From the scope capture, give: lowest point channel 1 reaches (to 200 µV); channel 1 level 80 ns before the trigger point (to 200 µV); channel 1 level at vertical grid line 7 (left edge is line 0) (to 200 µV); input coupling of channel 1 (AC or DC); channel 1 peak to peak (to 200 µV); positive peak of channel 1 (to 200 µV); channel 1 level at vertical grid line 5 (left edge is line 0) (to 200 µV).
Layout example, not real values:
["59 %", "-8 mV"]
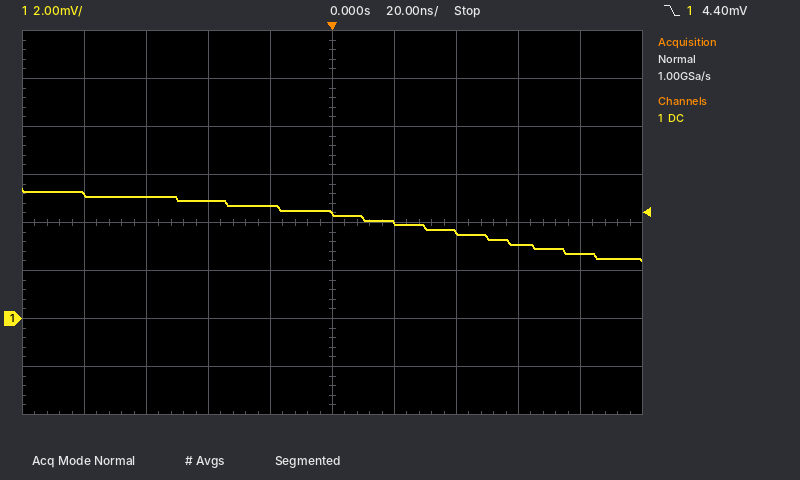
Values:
["2.4 mV", "5.2 mV", "3.6 mV", "DC", "3.0 mV", "5.4 mV", "4.4 mV"]
